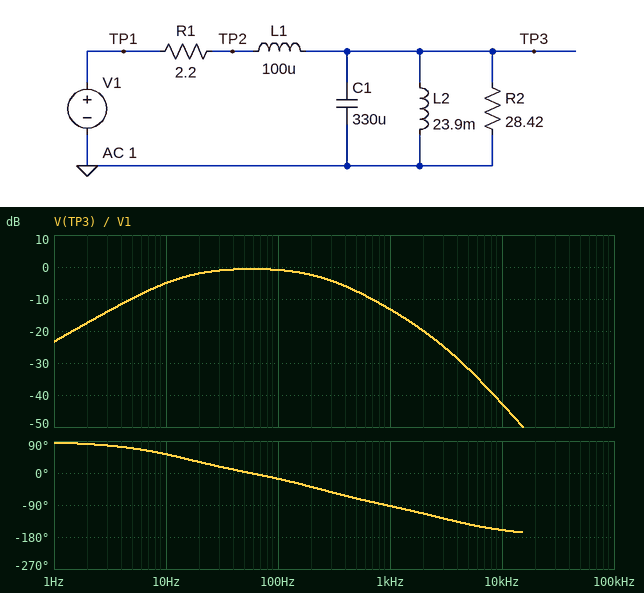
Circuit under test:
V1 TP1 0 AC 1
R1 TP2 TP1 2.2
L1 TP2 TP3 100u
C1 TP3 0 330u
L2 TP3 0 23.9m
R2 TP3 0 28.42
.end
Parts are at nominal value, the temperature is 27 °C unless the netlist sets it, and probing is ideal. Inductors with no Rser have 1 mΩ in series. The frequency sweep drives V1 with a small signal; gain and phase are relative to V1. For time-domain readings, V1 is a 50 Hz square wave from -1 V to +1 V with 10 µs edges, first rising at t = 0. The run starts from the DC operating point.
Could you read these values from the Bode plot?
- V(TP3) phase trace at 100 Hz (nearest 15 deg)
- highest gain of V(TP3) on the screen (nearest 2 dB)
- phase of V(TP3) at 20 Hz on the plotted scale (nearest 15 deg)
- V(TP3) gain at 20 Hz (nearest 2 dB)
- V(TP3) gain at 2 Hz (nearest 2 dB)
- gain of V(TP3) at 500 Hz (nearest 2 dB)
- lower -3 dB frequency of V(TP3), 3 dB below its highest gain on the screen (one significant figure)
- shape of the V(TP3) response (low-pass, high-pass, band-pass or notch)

-15 deg
0 dB
30 deg
-2 dB
-18 dB
-8 dB
10 Hz
band-pass
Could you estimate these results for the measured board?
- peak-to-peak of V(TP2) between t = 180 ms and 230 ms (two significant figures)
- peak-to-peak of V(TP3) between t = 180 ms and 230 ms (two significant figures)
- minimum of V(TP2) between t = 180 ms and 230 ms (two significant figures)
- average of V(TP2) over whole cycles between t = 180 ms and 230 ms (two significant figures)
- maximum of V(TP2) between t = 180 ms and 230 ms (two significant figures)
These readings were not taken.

2.4 V
2.3 V
-1.2 V
170 mV
1.2 V
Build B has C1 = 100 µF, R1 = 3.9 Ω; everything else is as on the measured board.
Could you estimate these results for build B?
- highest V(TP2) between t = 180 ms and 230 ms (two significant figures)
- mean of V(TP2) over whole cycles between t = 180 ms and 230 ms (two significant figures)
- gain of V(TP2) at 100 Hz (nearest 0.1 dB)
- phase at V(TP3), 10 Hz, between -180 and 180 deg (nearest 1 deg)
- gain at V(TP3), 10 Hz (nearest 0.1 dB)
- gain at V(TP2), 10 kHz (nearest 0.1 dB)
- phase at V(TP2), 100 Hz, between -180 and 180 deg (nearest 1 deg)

1.3 V
150 mV
-1.1 dB
66 deg
-9.0 dB
-1.5 dB
1 deg
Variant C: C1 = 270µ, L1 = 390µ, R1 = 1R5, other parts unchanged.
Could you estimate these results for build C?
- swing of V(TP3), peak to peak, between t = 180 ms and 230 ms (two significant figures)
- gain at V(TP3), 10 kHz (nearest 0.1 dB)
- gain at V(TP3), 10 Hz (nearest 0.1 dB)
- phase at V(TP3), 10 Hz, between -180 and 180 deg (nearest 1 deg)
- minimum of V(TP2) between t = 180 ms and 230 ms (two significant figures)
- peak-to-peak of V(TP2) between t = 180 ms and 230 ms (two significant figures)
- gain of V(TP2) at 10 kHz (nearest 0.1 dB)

2.7 V
-52.4 dB
-3.2 dB
42 deg
-1.3 V
2.5 V
0 dB
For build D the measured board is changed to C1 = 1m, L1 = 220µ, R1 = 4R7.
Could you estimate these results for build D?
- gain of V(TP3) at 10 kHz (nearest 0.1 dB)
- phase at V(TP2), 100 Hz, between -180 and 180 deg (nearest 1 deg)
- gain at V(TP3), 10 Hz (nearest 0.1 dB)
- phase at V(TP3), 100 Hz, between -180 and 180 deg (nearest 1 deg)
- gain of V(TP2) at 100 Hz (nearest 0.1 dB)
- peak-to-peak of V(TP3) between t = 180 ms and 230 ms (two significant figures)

-59.2 dB
-67 deg
-9.7 dB
-68 deg
-9.8 dB
1.6 V
